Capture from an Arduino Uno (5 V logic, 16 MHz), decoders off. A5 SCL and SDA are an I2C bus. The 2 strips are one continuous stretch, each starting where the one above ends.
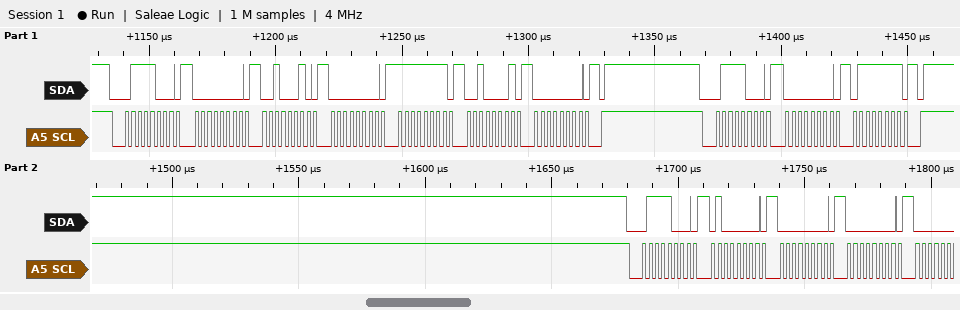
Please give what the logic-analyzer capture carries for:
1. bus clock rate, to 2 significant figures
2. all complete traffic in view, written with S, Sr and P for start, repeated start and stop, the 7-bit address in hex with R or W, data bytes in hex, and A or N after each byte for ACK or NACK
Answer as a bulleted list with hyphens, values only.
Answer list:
- 400 kHz
- S 3CW A 00 A 22 A 00 A FF A 21 A 00 A P S 3CW A 00 A 7F A P S 3CW A 40 A 00 A 00 A
